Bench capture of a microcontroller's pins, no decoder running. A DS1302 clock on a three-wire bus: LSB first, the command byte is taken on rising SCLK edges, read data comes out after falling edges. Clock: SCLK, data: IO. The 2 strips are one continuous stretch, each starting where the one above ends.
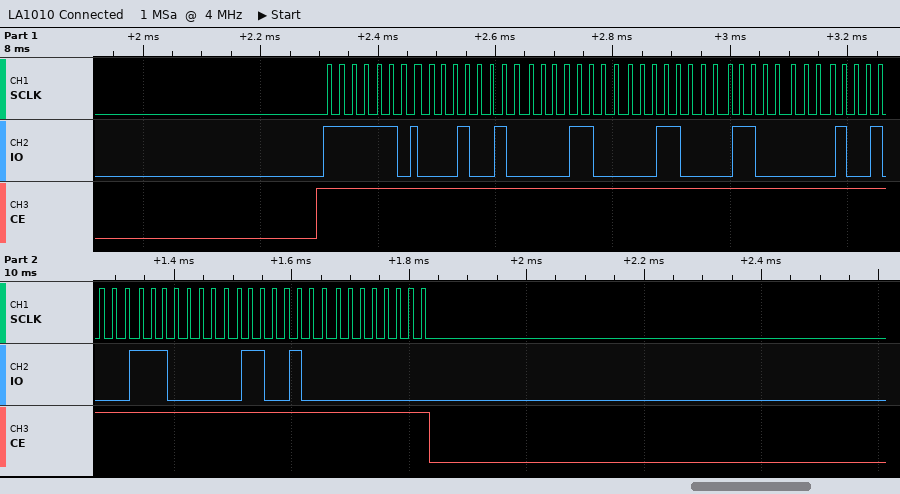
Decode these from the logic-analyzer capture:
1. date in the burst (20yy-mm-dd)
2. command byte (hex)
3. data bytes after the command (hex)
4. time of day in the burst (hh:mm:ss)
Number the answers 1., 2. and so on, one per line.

1. 2026-12-06
2. 0xBF
3. 48 30 18 06 12 07 26 00
4. 18:30:48
